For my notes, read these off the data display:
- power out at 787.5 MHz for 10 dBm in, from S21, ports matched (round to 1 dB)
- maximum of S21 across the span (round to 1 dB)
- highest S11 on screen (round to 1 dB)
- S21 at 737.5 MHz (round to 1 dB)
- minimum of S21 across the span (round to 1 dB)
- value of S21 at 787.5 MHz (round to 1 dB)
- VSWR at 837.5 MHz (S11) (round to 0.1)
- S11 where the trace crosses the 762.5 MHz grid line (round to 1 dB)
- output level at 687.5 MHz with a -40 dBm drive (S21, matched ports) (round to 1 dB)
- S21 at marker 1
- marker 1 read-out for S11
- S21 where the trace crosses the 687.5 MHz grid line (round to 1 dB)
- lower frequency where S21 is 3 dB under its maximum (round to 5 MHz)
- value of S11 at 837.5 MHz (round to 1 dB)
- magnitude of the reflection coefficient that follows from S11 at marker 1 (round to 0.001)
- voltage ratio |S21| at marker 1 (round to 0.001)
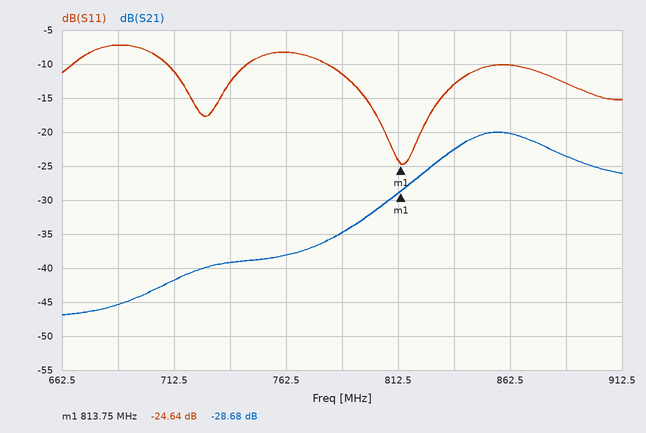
-25 dBm
-20 dB
-7 dB
-39 dB
-47 dB
-35 dB
1.6
-8 dB
-85 dBm
-28.68 dB
-24.64 dB
-45 dB
835 MHz
-13 dB
0.059
0.037
